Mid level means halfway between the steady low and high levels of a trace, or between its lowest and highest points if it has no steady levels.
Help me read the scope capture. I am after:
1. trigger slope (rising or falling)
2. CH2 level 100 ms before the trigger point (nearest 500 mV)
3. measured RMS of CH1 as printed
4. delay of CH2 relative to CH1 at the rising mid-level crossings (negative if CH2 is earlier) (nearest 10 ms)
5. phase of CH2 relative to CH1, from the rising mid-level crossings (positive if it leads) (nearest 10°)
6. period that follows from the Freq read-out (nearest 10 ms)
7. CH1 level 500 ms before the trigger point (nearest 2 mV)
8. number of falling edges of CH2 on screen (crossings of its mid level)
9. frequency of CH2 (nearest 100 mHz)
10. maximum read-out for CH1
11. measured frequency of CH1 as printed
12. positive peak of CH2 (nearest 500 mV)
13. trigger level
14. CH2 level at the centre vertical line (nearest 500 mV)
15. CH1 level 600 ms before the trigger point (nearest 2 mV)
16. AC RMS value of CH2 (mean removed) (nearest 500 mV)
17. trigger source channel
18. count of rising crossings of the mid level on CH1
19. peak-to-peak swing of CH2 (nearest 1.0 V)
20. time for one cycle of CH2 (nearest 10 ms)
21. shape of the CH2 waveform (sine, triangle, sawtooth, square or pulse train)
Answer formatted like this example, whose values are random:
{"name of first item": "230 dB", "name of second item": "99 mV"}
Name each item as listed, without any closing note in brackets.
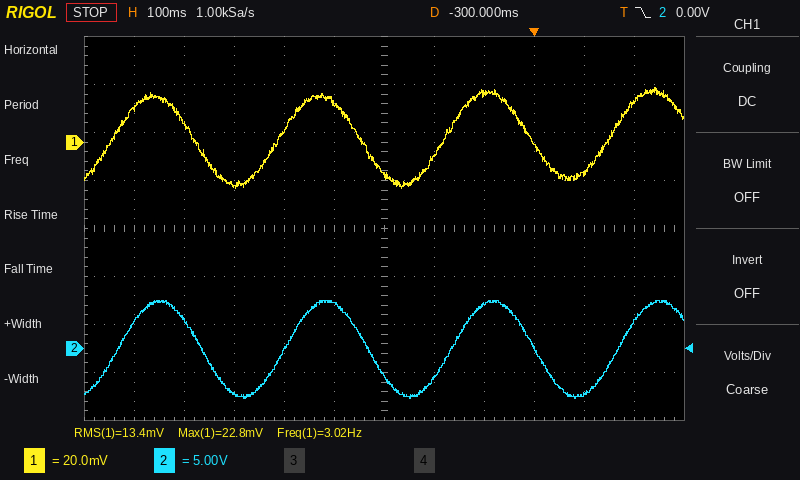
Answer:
{"trigger slope": "falling", "CH2 level 100 ms before the trigger point": "4.5 V", "measured RMS of CH1 as printed": "13.4 mV", "delay of CH2 relative to CH1 at the rising mid-level crossings (negative if CH2 is earlier)": "+10 ms", "phase of CH2 relative to CH1, from the rising mid-level crossings (positive if it leads)": "-10°", "period that follows from the Freq read-out": "330 ms", "CH1 level 500 ms before the trigger point": "4 mV", "number of falling edges of CH2 on screen": "3", "frequency of CH2": "3.0 Hz", "maximum read-out for CH1": "22.8 mV", "measured frequency of CH1 as printed": "3.02 Hz", "positive peak of CH2": "5.0 V", "trigger level": "0.00 V", "CH2 level at the centre vertical line": "-3.0 V", "CH1 level 600 ms before the trigger point": "-18 mV", "AC RMS value of CH2 (mean removed)": "3.5 V", "trigger source channel": "CH2", "count of rising crossings of the mid level on CH1": "4", "peak-to-peak swing of CH2": "10.0 V", "time for one cycle of CH2": "330 ms", "shape of the CH2 waveform": "sine"}
